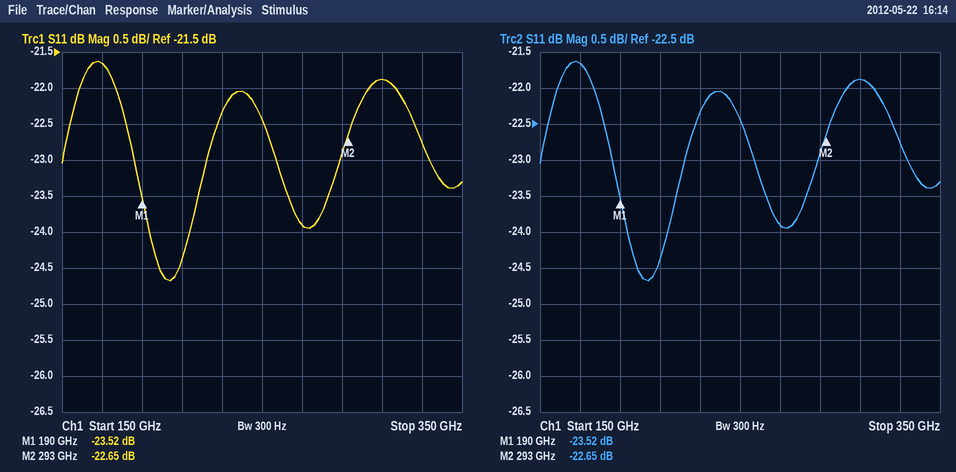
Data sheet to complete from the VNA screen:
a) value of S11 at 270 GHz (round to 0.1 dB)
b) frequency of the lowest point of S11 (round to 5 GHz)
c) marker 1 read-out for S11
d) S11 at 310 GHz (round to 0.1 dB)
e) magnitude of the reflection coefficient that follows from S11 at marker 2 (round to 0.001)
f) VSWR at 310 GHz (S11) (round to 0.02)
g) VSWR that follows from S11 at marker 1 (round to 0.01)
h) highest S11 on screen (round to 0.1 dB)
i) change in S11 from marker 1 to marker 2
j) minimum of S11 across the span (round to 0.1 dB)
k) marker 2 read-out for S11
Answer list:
-23.9 dB
205 GHz
-23.52 dB
-21.9 dB
0.074
1.18
1.14
-21.6 dB
0.87 dB
-24.7 dB
-22.65 dB
